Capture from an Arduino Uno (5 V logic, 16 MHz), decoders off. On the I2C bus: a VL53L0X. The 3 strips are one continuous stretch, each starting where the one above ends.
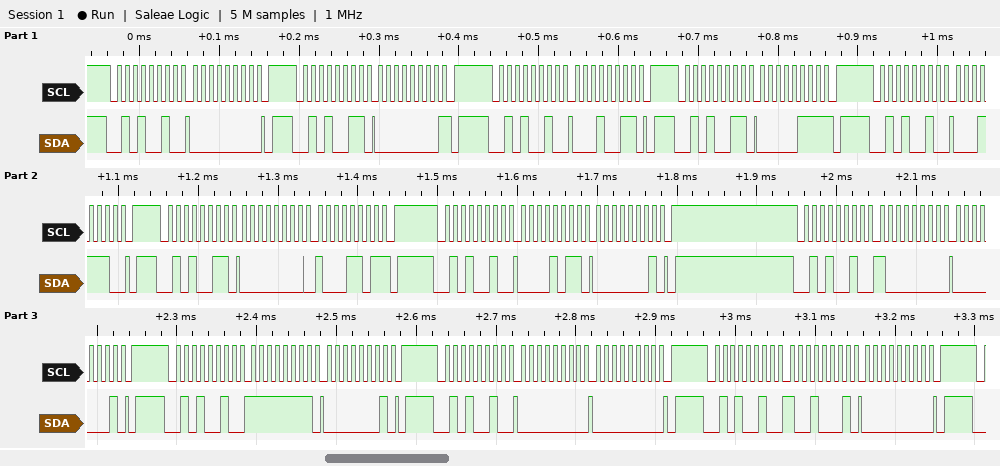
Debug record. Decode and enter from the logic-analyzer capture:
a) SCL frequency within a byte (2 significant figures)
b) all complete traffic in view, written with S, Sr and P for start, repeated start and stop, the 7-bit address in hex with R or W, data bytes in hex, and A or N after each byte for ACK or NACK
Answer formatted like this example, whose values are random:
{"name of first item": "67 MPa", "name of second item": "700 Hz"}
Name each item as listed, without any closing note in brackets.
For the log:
{"SCL frequency within a byte": "100 kHz", "all complete traffic in view, written with S, Sr and P for start, repeated start and stop, the 7-bit address in hex with R or W, data bytes in hex, and A or N after each byte for ACK or NACK": "S 29W A 00 A P S 29R A 00 N P S 29W A 13 A P S 29R A 07 N P S 29W A 1E A P S 29R A 00 A 8D N P S 29W A 0B A 01 A P S 29W A 80 A 01 A P S 29W A FF A 01 A P S 29W A 00 A 00 A P S 29W A 91 A 00 A P"}
